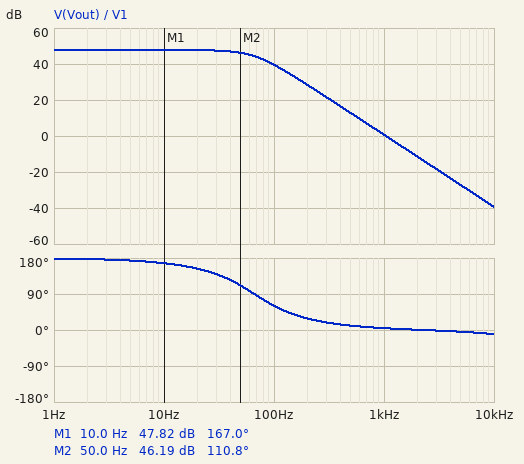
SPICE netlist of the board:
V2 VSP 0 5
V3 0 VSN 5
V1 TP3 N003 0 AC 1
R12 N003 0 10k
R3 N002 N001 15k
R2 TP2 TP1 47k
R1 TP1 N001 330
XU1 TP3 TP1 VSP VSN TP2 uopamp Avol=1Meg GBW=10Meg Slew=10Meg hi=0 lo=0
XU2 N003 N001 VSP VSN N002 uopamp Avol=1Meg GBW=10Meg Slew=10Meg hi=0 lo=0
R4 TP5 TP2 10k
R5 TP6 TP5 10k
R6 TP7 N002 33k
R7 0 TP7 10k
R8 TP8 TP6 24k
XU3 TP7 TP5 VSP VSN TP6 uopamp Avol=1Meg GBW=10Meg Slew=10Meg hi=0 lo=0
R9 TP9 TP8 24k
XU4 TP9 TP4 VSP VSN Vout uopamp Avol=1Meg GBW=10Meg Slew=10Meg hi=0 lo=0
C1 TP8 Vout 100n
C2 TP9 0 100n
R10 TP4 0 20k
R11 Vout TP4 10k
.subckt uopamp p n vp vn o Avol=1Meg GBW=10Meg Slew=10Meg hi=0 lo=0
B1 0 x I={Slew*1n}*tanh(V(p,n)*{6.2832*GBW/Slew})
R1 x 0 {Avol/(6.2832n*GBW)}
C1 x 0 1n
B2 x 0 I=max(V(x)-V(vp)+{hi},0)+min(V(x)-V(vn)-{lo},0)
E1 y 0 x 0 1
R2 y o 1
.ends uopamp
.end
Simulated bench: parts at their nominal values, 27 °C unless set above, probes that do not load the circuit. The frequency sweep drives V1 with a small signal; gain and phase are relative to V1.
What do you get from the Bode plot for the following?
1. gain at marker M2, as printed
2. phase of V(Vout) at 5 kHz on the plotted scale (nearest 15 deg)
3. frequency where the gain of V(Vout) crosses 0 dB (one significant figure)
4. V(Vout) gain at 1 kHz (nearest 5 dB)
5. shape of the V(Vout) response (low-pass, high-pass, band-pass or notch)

46.19 dB
0 deg
1 kHz
0 dB
low-pass
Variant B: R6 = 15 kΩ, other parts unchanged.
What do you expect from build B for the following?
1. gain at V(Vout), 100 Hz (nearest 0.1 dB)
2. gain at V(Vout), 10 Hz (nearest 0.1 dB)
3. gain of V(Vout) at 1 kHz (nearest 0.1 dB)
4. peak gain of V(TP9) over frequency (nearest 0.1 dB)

40.3 dB
48.6 dB
1.5 dB
45.1 dB
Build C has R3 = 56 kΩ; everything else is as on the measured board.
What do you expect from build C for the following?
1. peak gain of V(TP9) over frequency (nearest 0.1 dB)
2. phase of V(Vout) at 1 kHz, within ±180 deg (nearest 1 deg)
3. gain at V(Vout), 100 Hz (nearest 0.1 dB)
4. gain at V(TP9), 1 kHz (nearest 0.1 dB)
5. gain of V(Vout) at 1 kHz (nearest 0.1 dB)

46.9 dB
4 deg
42.2 dB
-0.2 dB
3.3 dB
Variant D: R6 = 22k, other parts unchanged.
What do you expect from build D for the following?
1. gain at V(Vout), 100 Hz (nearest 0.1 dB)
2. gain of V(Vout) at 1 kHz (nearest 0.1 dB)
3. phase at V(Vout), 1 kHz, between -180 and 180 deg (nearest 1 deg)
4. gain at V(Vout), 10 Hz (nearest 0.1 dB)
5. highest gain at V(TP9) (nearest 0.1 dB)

39.9 dB
1.1 dB
5 deg
48.2 dB
44.7 dB
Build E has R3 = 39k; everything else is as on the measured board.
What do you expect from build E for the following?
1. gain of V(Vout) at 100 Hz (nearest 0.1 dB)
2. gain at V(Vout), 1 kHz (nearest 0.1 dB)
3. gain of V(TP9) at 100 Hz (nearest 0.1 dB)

41.2 dB
2.3 dB
37.7 dB
